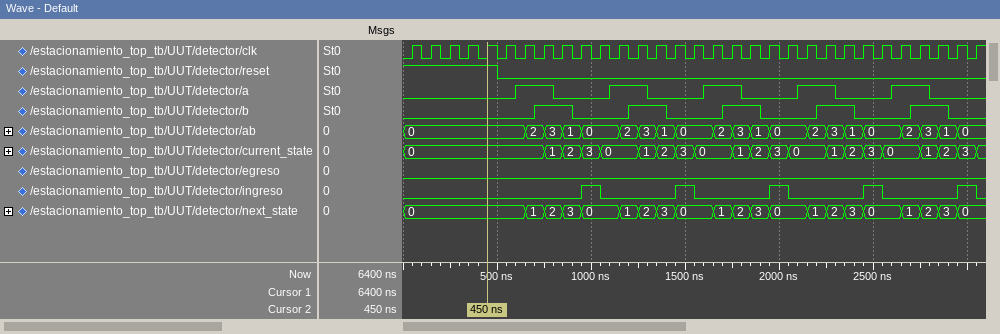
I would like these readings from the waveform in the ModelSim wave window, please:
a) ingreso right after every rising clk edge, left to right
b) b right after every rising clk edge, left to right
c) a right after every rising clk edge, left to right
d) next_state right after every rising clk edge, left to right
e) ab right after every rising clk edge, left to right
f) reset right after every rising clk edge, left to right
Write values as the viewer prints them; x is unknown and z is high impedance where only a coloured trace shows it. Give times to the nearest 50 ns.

0 0 0 0 0 0 0 0 0 1 0 0 0 0 1 0 0 0 0 1 0 0 0 0 1 0 0 0 0 1 0
0 0 0 0 0 0 0 1 1 0 0 0 1 1 0 0 0 1 1 0 0 0 1 1 0 0 0 1 1 0 0
0 0 0 0 0 0 1 1 0 0 0 1 1 0 0 0 1 1 0 0 0 1 1 0 0 0 1 1 0 0 0
0, 0, 0, 0, 0, 0, 1, 2, 3, 0, 0, 1, 2, 3, 0, 0, 1, 2, 3, 0, 0, 1, 2, 3, 0, 0, 1, 2, 3, 0, 0
0, 0, 0, 0, 0, 0, 2, 3, 1, 0, 0, 2, 3, 1, 0, 0, 2, 3, 1, 0, 0, 2, 3, 1, 0, 0, 2, 3, 1, 0, 0
1 1 1 1 1 0 0 0 0 0 0 0 0 0 0 0 0 0 0 0 0 0 0 0 0 0 0 0 0 0 0
